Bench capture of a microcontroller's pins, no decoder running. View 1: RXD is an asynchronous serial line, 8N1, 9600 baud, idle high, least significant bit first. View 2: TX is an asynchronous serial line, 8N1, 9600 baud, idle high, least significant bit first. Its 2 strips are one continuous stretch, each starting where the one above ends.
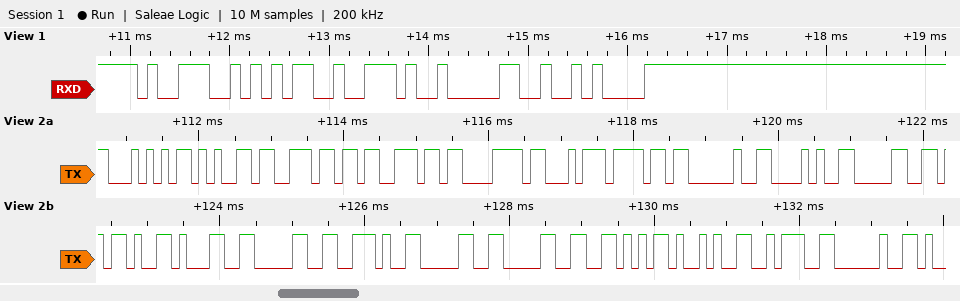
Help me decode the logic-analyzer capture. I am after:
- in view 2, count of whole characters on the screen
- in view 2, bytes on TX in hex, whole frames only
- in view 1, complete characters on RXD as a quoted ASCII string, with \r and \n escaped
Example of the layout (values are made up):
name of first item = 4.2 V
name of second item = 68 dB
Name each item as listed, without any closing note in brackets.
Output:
in view 2, count of whole characters on the screen = 20
in view 2, bytes on TX in hex, whole frames only = 54 65 6E 73 C3 A3 6F 20 28 30 2D 31 30 2E 30 30 56 29 3A 20
in view 1, complete characters on RXD as a quoted ASCII string, with \r and \n escaped = "95.0\n"
